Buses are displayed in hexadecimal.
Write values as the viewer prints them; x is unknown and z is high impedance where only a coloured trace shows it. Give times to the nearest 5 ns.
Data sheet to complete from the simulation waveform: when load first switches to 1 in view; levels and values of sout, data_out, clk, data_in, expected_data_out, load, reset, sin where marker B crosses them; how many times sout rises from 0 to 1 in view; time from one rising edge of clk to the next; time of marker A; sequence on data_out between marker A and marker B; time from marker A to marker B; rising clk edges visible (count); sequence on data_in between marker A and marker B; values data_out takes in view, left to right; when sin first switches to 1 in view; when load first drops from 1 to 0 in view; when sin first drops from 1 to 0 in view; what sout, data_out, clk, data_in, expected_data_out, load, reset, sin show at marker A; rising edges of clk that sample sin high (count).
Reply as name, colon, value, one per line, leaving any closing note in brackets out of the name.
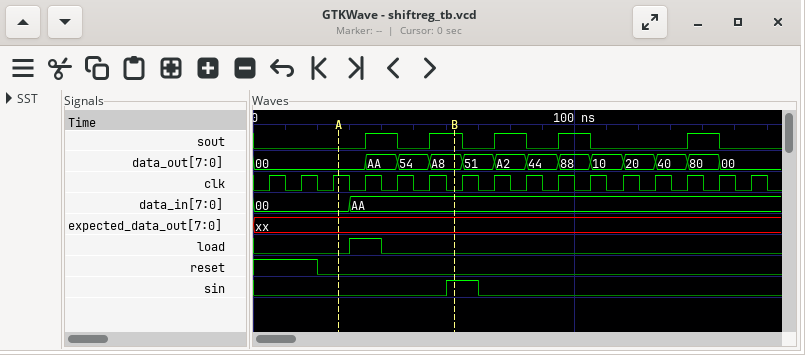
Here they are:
when load first switches to 1 in view: 30 ns
levels and values of sout, data_out, clk, data_in, expected_data_out, load, reset, sin where marker B crosses them: sout=1, data_out=A8, clk=0, data_in=AA, expected_data_out=xx, load=0, reset=0, sin=1
how many times sout rises from 0 to 1 in view: 5
time from one rising edge of clk to the next: 10 ns
time of marker A: 25 ns
sequence on data_out between marker A and marker B: 00, AA, 54, A8
time from marker A to marker B: 35 ns
rising clk edges visible: 16
sequence on data_in between marker A and marker B: 00, AA
values data_out takes in view, left to right: 00, AA, 54, A8, 51, A2, 44, 88, 10, 20, 40, 80, 00
when sin first switches to 1 in view: 60 ns
when load first drops from 1 to 0 in view: 40 ns
when sin first drops from 1 to 0 in view: 70 ns
what sout, data_out, clk, data_in, expected_data_out, load, reset, sin show at marker A: sout=0, data_out=00, clk=1, data_in=00, expected_data_out=xx, load=0, reset=0, sin=0
rising edges of clk that sample sin high: 1
